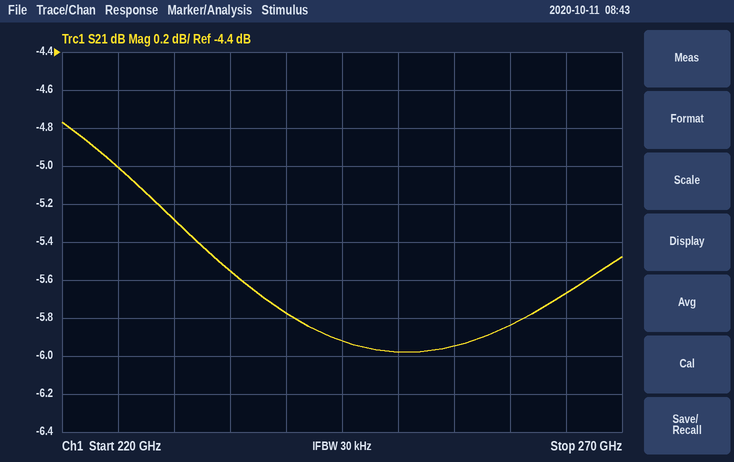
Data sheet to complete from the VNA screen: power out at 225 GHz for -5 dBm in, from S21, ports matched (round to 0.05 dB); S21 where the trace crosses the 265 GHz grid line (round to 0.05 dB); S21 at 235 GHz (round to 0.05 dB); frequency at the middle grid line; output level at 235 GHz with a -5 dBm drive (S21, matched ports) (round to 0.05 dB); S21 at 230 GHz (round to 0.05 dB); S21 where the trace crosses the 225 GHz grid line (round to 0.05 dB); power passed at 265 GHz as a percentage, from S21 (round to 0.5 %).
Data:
-10.00 dBm
-5.65 dB
-5.55 dB
245 GHz
-10.55 dBm
-5.30 dB
-5.00 dB
27.0 %
